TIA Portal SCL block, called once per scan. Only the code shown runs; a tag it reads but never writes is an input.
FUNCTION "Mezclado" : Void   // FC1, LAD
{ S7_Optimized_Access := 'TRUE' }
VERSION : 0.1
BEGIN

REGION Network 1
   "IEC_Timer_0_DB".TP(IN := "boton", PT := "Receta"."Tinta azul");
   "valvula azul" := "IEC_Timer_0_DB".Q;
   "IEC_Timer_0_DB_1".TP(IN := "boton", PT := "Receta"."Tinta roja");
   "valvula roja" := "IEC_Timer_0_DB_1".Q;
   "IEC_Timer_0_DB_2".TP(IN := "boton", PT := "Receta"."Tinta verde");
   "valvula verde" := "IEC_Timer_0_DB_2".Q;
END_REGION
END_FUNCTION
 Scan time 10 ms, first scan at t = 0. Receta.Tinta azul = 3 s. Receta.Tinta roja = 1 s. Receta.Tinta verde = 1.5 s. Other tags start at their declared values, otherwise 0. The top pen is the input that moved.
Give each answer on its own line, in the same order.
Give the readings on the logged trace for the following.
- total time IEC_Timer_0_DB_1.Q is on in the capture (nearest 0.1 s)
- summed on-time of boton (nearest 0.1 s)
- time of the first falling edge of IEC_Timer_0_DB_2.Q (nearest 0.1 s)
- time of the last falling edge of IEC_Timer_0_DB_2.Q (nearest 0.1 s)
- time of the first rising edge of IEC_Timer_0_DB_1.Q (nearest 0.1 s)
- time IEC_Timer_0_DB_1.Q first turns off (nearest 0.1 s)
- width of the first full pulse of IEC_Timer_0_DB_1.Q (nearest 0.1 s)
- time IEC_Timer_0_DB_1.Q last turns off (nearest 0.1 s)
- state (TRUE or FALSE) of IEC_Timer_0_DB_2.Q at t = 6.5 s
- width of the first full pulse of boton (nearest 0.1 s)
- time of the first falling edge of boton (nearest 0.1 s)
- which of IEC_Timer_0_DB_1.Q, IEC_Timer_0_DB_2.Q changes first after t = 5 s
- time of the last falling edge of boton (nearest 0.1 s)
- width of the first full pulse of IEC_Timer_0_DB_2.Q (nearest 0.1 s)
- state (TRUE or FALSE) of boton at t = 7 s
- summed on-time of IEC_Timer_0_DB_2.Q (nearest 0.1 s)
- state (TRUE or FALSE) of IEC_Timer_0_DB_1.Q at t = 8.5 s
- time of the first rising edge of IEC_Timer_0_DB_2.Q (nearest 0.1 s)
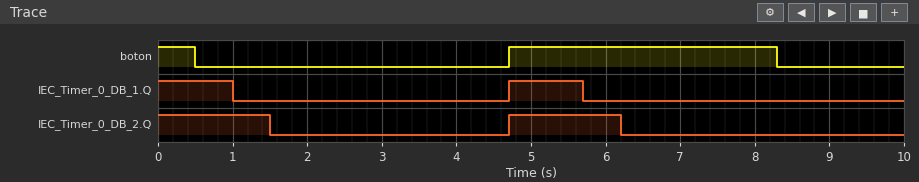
2.0 s
4.1 s
1.5 s
6.2 s
4.7 s
1.0 s
1.0 s
5.7 s
FALSE
3.6 s
0.5 s
IEC_Timer_0_DB_1.Q
8.3 s
1.5 s
TRUE
3.0 s
FALSE
4.7 s
